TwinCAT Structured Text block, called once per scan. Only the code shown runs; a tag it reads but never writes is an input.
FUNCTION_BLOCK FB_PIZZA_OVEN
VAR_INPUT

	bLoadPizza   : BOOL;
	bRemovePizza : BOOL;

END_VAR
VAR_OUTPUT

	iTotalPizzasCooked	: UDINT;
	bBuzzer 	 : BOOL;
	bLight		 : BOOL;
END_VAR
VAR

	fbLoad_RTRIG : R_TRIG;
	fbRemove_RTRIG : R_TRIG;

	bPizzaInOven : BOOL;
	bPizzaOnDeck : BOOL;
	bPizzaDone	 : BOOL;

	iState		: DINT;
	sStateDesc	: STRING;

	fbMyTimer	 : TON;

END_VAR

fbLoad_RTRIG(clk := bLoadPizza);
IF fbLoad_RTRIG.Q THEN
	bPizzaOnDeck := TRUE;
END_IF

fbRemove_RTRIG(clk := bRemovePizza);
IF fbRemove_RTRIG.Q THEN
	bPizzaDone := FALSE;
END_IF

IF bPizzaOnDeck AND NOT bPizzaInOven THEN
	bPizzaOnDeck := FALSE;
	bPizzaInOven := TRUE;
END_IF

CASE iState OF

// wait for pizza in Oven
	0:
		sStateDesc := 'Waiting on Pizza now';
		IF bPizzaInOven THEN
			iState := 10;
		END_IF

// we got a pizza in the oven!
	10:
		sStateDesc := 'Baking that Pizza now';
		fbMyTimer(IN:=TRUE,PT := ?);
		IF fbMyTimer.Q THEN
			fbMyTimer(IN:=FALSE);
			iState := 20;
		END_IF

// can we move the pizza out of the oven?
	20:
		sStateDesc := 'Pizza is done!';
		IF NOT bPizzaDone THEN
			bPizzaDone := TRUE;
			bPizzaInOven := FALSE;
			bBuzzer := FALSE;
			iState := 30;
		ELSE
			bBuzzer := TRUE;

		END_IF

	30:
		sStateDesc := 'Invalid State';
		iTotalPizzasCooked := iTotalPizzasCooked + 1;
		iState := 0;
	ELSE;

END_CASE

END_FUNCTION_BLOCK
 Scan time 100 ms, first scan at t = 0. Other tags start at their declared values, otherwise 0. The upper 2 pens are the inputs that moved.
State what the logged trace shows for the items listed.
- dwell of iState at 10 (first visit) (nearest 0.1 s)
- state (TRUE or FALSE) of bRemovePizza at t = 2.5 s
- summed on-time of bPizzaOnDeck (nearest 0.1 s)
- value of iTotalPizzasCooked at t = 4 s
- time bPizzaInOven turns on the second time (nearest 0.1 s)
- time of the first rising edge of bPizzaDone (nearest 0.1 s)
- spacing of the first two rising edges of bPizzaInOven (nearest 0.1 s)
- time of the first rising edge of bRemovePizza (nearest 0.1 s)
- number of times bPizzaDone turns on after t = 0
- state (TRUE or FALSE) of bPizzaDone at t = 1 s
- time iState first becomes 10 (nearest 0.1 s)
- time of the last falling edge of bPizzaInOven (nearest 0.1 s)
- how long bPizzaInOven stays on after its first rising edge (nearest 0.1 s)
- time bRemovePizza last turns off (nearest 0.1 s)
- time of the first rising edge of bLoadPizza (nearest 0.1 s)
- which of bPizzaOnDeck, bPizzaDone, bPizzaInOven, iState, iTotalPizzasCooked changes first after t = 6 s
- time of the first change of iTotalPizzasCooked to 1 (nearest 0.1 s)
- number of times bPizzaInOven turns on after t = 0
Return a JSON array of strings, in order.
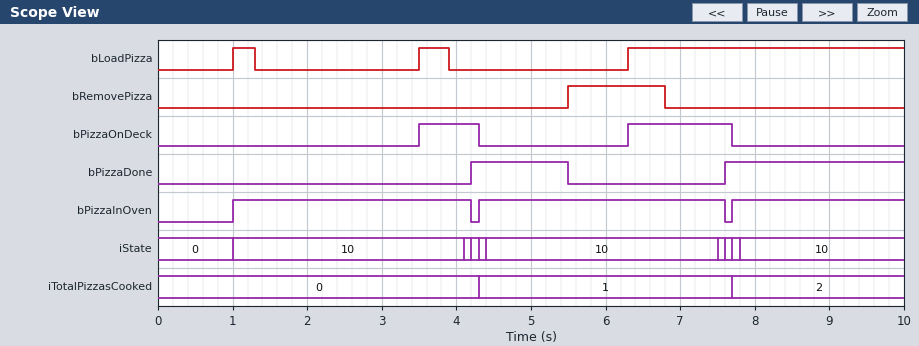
["3.1 s", "FALSE", "2.2 s", "0", "4.3 s", "4.2 s", "3.3 s", "5.5 s", "2", "FALSE", "1.0 s", "7.6 s", "3.2 s", "6.8 s", "1.0 s", "bPizzaOnDeck", "4.3 s", "3"]
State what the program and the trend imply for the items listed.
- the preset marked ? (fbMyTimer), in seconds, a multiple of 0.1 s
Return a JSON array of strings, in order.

["3.0 s"]
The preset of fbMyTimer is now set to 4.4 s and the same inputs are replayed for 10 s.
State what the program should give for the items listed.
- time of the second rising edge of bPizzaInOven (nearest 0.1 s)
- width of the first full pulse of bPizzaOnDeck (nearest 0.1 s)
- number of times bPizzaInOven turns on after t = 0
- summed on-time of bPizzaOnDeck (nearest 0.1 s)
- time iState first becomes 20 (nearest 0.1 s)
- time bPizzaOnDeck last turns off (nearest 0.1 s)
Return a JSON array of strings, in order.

["5.7 s", "2.2 s", "2", "5.9 s", "5.5 s", "5.7 s"]
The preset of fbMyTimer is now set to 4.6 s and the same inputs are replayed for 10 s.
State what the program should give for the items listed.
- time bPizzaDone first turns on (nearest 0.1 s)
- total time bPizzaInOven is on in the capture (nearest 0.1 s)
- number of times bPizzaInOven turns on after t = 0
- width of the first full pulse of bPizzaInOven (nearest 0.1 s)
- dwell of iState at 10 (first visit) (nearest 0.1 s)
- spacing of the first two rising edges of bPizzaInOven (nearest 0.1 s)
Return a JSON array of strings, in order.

["5.8 s", "8.9 s", "2", "4.8 s", "4.7 s", "4.9 s"]
